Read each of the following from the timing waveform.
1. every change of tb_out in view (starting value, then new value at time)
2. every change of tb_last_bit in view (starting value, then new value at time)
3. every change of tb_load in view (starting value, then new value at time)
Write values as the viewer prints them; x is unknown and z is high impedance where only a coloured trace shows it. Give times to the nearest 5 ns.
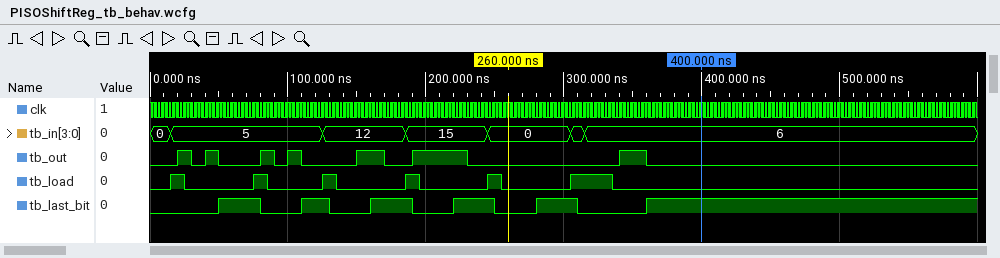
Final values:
0, 1 at 20 ns, 0 at 30 ns, 1 at 40 ns, 0 at 50 ns, 1 at 80 ns, 0 at 90 ns, 1 at 100 ns, 0 at 110 ns, 1 at 150 ns, 0 at 170 ns, 1 at 190 ns, 0 at 230 ns, 1 at 340 ns, 0 at 360 ns
0, 1 at 50 ns, 0 at 80 ns, 1 at 110 ns, 0 at 130 ns, 1 at 160 ns, 0 at 190 ns, 1 at 220 ns, 0 at 250 ns, 1 at 280 ns, 0 at 310 ns, 1 at 360 ns
0, 1 at 15 ns, 0 at 25 ns, 1 at 75 ns, 0 at 85 ns, 1 at 125 ns, 0 at 135 ns, 1 at 185 ns, 0 at 195 ns, 1 at 245 ns, 0 at 255 ns, 1 at 305 ns, 0 at 335 ns
